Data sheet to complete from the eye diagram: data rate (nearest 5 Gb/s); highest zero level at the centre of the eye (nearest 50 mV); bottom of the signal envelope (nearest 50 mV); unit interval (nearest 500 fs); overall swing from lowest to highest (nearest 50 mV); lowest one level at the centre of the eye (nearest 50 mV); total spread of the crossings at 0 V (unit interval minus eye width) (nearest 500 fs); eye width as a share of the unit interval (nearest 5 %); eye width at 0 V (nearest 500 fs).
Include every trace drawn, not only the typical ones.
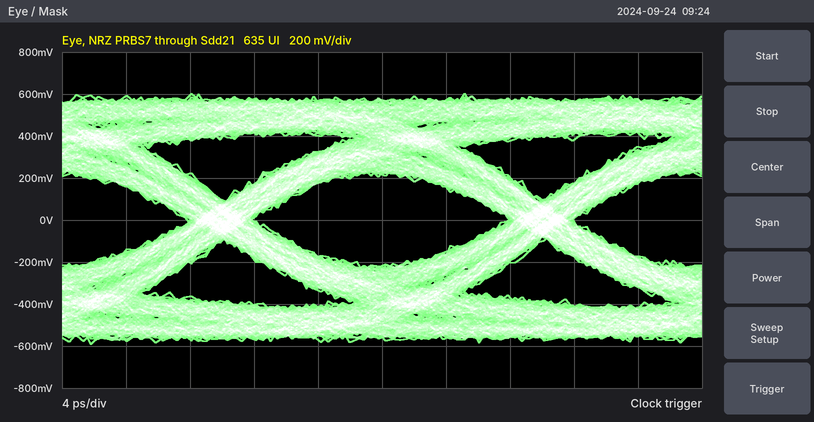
50 Gb/s
-200 mV
-600 mV
20.0 ps
1.20 V
200 mV
4.0 ps
80 %
16.0 ps
